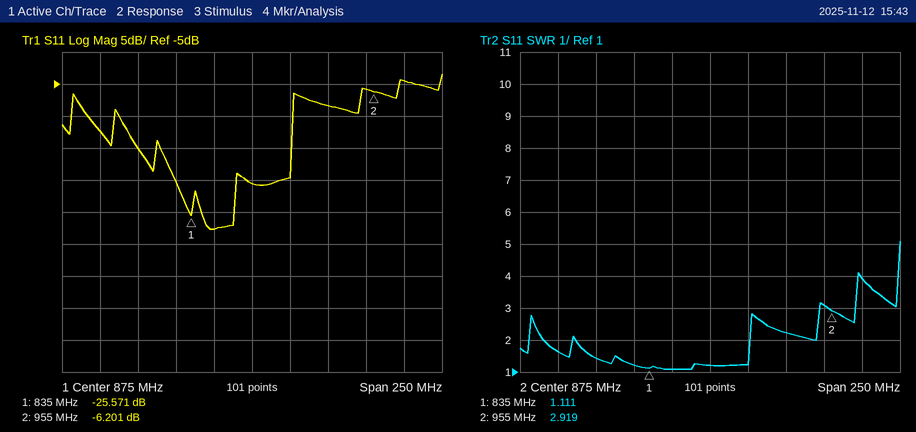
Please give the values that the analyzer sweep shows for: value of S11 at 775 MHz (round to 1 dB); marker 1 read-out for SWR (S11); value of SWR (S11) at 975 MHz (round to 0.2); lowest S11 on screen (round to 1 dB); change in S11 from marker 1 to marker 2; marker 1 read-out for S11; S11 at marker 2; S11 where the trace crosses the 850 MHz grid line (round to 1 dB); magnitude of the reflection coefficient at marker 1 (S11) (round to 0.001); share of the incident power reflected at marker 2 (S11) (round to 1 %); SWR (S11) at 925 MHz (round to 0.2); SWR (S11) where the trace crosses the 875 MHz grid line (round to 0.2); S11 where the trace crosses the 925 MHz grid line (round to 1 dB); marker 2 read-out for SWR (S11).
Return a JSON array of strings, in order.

["-12 dB", "1.111", "4.0", "-28 dB", "19.370 dB", "-25.571 dB", "-6.201 dB", "-28 dB", "0.053", "24 %", "2.2", "1.2", "-8 dB", "2.919"]
